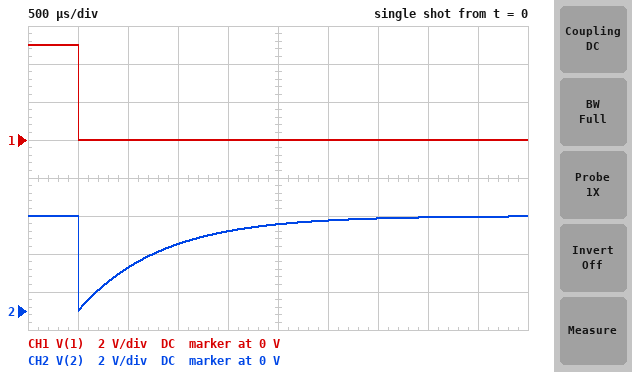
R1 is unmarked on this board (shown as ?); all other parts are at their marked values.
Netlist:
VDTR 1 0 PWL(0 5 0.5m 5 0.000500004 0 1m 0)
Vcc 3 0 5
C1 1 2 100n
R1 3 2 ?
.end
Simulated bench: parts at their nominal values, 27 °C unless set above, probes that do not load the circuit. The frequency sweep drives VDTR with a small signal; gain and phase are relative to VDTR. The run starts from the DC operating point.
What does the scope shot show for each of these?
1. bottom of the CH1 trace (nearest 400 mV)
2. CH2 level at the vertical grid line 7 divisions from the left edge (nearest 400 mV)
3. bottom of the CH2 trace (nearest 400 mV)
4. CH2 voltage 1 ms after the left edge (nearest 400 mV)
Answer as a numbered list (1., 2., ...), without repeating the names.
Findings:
1. 0 V
2. 4.8 V
3. 0 V
4. 2.4 V
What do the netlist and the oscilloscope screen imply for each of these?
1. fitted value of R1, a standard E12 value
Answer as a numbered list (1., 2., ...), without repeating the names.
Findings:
1. 8.2 kΩ
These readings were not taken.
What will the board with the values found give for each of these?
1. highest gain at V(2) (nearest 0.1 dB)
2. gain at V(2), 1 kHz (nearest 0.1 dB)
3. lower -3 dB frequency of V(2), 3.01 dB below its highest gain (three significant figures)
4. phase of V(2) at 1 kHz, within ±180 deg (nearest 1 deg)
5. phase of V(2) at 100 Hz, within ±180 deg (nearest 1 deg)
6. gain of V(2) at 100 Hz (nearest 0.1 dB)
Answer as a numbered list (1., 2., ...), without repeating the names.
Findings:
1. 0 dB
2. -0.2 dB
3. 194 Hz
4. 11 deg
5. 63 deg
6. -6.8 dB
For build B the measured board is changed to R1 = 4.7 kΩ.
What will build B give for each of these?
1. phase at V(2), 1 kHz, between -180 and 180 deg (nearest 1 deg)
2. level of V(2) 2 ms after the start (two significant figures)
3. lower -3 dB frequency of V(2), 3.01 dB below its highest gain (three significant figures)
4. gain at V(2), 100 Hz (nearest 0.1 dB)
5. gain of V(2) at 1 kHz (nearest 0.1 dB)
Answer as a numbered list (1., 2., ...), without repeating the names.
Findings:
1. 19 deg
2. 4.8 V
3. 339 Hz
4. -11.0 dB
5. -0.5 dB
